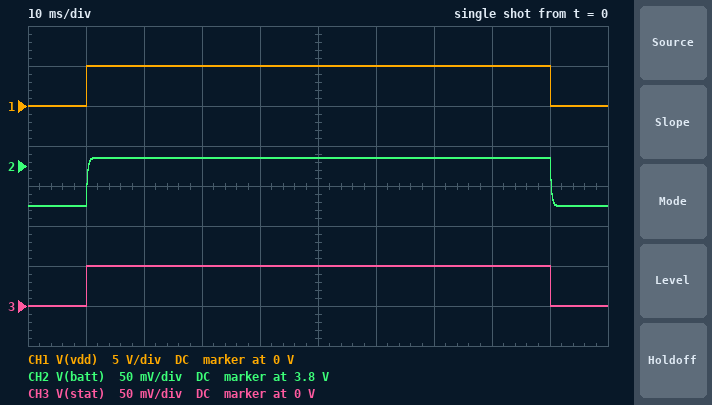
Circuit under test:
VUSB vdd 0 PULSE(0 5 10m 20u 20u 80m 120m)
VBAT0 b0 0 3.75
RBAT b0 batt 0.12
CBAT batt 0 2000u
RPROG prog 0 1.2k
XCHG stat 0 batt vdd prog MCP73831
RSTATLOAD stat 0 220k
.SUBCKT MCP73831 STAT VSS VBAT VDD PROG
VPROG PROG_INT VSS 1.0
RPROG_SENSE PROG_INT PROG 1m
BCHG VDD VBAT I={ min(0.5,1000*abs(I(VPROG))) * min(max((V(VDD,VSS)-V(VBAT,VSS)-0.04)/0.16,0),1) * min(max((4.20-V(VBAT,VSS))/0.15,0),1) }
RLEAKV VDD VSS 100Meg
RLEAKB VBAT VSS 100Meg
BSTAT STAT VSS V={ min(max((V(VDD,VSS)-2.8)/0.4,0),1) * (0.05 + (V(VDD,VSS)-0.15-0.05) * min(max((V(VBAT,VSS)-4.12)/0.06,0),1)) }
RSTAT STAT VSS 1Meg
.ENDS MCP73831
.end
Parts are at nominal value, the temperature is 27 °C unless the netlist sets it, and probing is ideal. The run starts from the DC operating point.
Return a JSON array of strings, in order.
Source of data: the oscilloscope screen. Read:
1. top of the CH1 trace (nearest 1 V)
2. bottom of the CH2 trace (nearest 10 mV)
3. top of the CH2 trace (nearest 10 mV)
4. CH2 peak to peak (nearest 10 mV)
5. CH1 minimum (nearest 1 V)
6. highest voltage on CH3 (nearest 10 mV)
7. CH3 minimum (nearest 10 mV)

["5 V", "3.75 V", "3.81 V", "60 mV", "0 V", "50 mV", "0 V"]
